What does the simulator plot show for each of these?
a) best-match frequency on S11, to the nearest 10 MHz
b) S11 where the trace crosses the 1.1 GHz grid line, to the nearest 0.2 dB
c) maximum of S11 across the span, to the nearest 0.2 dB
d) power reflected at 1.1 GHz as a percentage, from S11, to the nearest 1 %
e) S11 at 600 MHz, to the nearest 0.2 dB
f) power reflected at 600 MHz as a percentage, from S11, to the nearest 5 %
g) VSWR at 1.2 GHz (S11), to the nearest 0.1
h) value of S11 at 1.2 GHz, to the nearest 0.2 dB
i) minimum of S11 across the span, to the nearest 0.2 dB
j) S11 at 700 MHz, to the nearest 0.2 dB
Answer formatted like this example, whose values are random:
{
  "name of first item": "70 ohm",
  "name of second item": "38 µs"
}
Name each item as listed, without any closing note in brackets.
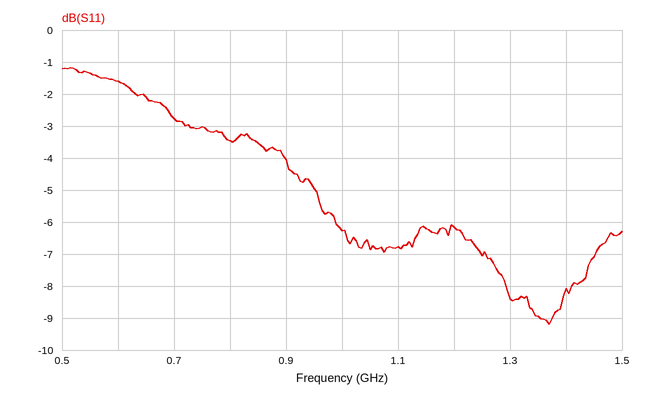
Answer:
{
  "best-match frequency on S11, to the nearest 10 MHz": "1.37 GHz",
  "S11 where the trace crosses the 1.1 GHz grid line, to the nearest 0.2 dB": "-6.8 dB",
  "maximum of S11 across the span, to the nearest 0.2 dB": "-1.2 dB",
  "power reflected at 1.1 GHz as a percentage, from S11, to the nearest 1 %": "21 %",
  "S11 at 600 MHz, to the nearest 0.2 dB": "-1.6 dB",
  "power reflected at 600 MHz as a percentage, from S11, to the nearest 5 %": "70 %",
  "VSWR at 1.2 GHz (S11), to the nearest 0.1": "2.9",
  "value of S11 at 1.2 GHz, to the nearest 0.2 dB": "-6.2 dB",
  "minimum of S11 across the span, to the nearest 0.2 dB": "-9.2 dB",
  "S11 at 700 MHz, to the nearest 0.2 dB": "-2.8 dB"
}
